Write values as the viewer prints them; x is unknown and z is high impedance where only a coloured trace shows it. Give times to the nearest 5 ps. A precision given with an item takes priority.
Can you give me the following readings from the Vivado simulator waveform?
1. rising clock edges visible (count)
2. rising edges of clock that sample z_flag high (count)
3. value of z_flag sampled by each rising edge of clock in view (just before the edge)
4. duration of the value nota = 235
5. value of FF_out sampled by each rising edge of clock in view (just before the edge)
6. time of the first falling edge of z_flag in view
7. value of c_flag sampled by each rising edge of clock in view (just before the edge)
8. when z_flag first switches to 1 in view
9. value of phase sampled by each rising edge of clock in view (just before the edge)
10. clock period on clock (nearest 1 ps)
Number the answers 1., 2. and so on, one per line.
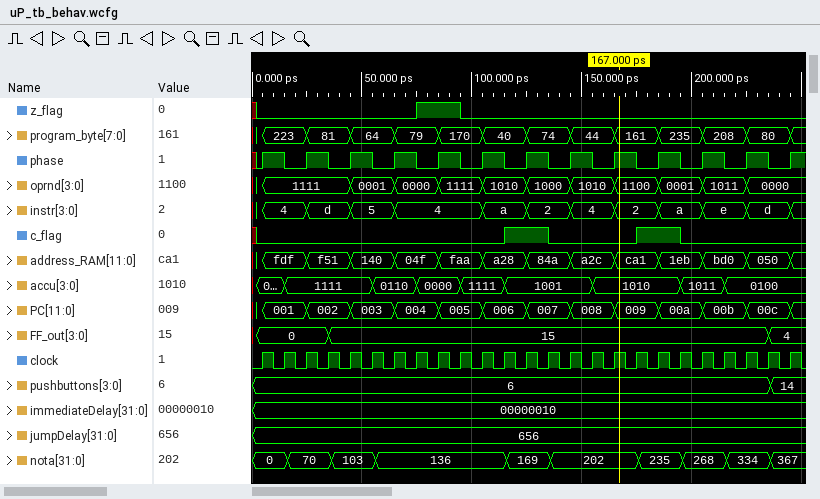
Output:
1. 25
2. 2
3. 0 0 0 0 0 0 0 0 1 1 0 0 0 0 0 0 0 0 0 0 0 0 0 0 0
4. 20 ps
5. 0, 0, 0, 0, 15, 15, 15, 15, 15, 15, 15, 15, 15, 15, 15, 15, 15, 15, 15, 15, 15, 15, 15, 15, 4
6. 95 ps
7. 0 0 0 0 0 0 0 0 0 0 0 0 1 1 0 0 0 0 1 1 0 0 0 0 0
8. 75 ps
9. 0 1 0 1 0 1 0 1 0 1 0 1 0 1 0 1 0 1 0 1 0 1 0 1 0
10. 10 ps
